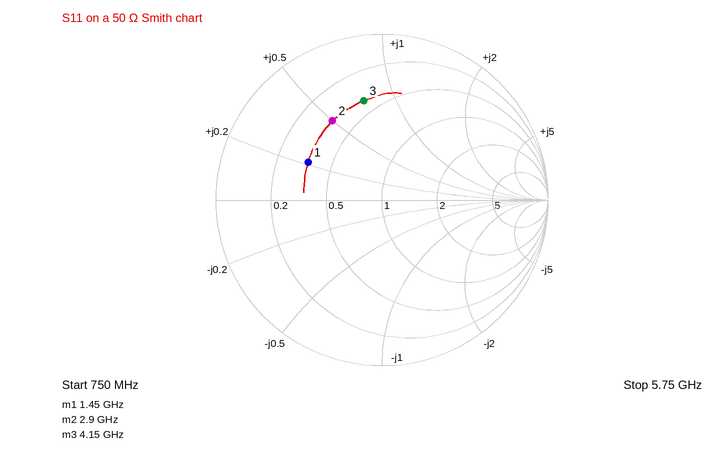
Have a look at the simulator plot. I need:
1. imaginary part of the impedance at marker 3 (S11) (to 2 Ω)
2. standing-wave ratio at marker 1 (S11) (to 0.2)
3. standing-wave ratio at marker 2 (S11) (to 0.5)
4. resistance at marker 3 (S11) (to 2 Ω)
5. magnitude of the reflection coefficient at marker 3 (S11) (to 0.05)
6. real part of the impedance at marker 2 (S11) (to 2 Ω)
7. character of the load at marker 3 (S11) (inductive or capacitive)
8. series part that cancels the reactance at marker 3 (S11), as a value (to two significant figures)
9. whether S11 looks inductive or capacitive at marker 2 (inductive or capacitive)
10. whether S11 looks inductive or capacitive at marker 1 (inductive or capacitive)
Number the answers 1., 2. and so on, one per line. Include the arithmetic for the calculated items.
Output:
1. +38 Ω
2. 3.0
3. 3.5
4. 20 Ω
5. 0.60
6. 18 Ω
7. inductive
8. C = 1/(2π × 4.15 GHz × 38 Ω) ≈ 1.0 pF
9. inductive
10. inductive
